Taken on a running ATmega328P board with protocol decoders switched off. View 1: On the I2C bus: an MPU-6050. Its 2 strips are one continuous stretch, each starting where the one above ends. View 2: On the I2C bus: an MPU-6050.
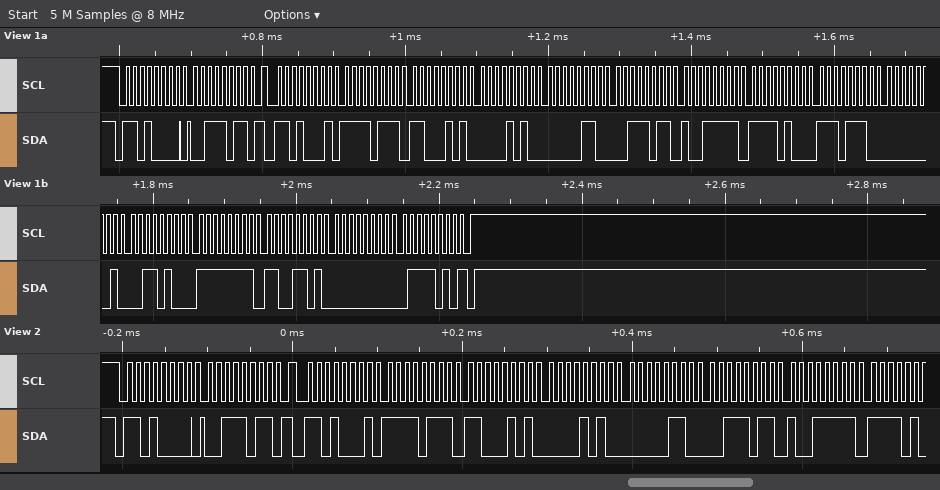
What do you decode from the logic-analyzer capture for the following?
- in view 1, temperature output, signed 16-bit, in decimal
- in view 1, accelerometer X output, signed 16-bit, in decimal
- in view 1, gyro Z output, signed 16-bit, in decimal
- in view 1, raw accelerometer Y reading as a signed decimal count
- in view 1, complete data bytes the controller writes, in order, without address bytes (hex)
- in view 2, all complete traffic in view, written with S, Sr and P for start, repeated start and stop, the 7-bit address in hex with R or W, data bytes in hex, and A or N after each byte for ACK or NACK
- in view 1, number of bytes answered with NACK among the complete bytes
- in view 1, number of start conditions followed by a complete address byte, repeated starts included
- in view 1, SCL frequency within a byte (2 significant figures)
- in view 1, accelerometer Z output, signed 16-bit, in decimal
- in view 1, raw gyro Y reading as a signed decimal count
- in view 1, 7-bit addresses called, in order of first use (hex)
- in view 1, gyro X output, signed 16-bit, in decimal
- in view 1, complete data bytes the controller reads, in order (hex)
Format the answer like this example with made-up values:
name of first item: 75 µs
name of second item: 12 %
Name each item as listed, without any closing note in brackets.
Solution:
in view 1, temperature output, signed 16-bit, in decimal: -2834
in view 1, accelerometer X output, signed 16-bit, in decimal: -2107
in view 1, gyro Z output, signed 16-bit, in decimal: 122
in view 1, raw accelerometer Y reading as a signed decimal count: 2566
in view 1, complete data bytes the controller writes, in order, without address bytes: 3B
in view 2, all complete traffic in view, written with S, Sr and P for start, repeated start and stop, the 7-bit address in hex with R or W, data bytes in hex, and A or N after each byte for ACK or NACK: S 68W A 3B A Sr 68R A F7 A C5 A 0A A 06 A 3B A 9F A
in view 1, number of bytes answered with NACK among the complete bytes: 1
in view 1, number of start conditions followed by a complete address byte, repeated starts included: 2
in view 1, SCL frequency within a byte: 100 kHz
in view 1, accelerometer Z output, signed 16-bit, in decimal: 15263
in view 1, raw gyro Y reading as a signed decimal count: -51
in view 1, 7-bit addresses called, in order of first use: 0x68
in view 1, gyro X output, signed 16-bit, in decimal: 308
in view 1, complete data bytes the controller reads, in order: F7 C5 0A 06 3B 9F F4 EE 01 34 FF CD 00 7A
